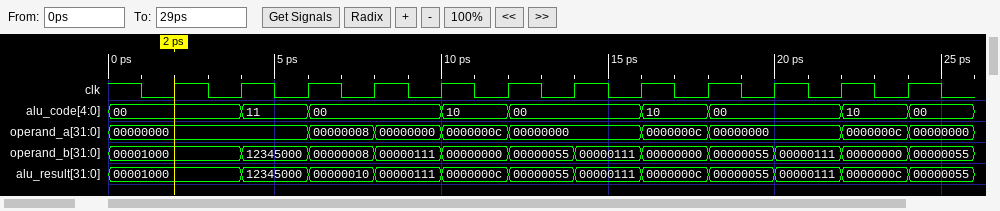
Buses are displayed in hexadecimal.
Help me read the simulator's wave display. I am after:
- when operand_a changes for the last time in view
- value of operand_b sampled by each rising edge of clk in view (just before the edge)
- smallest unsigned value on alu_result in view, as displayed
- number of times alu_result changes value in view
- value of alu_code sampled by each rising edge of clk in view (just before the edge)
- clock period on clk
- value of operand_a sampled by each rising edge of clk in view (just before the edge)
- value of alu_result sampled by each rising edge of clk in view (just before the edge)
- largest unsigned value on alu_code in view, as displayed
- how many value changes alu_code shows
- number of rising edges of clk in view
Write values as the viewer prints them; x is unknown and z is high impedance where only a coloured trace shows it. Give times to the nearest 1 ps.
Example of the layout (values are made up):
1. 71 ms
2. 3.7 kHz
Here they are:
1. 24 ps
2. 00001000, 00001000, 12345000, 00000008, 00000111, 00000000, 00000055, 00000111, 00000000, 00000055, 00000111, 00000000
3. 0000000c
4. 11
5. 00, 00, 11, 00, 00, 10, 00, 00, 10, 00, 00, 10
6. 2 ps
7. 00000000, 00000000, 00000000, 00000008, 00000000, 0000000c, 00000000, 00000000, 0000000c, 00000000, 00000000, 0000000c
8. 00001000, 00001000, 12345000, 00000010, 00000111, 0000000c, 00000055, 00000111, 0000000c, 00000055, 00000111, 0000000c
9. 11
10. 8
11. 12
